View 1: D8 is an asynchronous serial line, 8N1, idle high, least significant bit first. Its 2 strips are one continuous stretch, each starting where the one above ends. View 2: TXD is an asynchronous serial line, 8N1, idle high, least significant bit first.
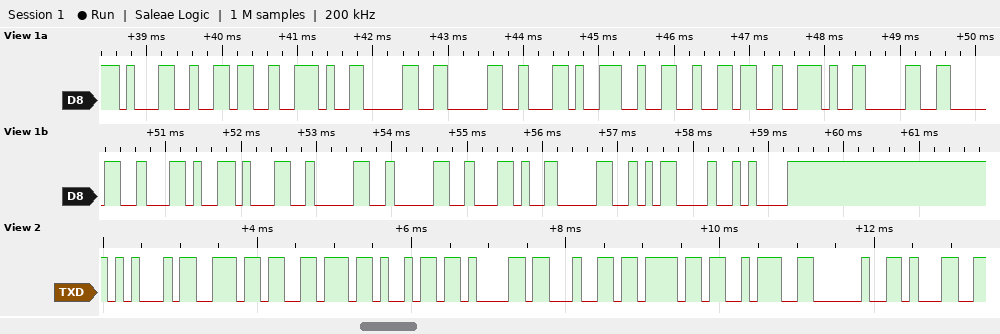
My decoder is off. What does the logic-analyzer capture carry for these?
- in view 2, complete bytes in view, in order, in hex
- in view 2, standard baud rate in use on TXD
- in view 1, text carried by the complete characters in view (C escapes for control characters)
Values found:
45 6E 76 69 61 64 6F 3A 20 31
9600 baud
"16.00,26.00,100,0\r\n"
